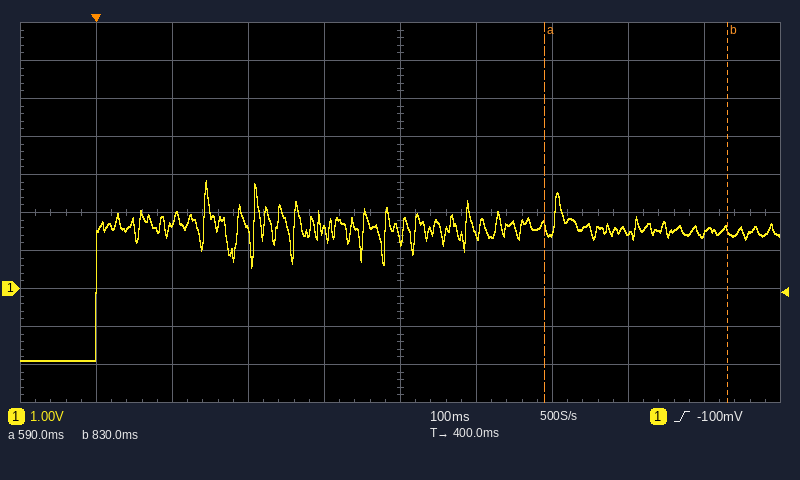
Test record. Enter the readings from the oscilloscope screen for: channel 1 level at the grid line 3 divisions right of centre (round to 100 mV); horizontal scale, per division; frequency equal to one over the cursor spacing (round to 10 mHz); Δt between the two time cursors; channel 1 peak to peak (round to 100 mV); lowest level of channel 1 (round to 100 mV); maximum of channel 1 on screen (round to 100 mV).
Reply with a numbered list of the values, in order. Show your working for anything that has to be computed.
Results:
1. 1.5 V
2. 100 ms
3. 1 / 240 ms ≈ 4.17 Hz
4. 830 ms − (590 ms) = 240 ms
5. 2.8 V − (-1.9 V) = 4.7 V
6. -1.9 V
7. 2.8 V
